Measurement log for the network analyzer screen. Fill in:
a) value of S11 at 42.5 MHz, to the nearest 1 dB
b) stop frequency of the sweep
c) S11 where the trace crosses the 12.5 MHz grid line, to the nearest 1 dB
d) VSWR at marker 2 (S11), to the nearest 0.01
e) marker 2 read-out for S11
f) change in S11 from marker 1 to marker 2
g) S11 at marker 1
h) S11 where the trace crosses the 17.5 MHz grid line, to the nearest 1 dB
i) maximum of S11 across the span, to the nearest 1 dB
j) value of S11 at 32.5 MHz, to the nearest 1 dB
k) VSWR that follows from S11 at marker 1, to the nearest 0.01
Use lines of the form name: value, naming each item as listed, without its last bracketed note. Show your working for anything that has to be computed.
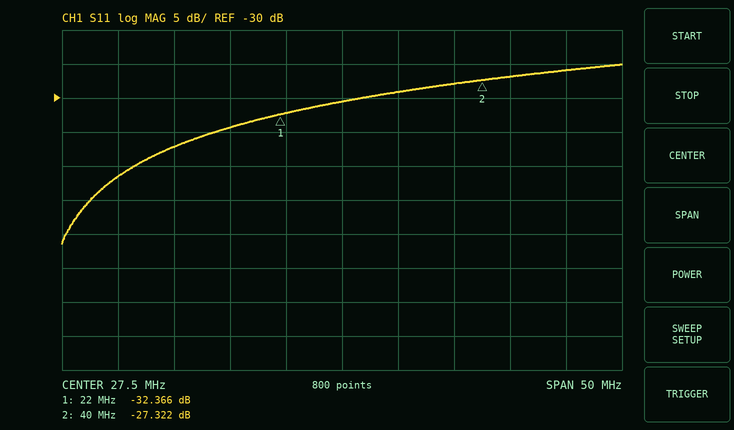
value of S11 at 42.5 MHz, to the nearest 1 dB: -27 dB
stop frequency of the sweep: 52.5 MHz
S11 where the trace crosses the 12.5 MHz grid line, to the nearest 1 dB: -37 dB
VSWR at marker 2 (S11), to the nearest 0.01: (1 + 0.0430)/(1 − 0.0430) ≈ 1.09
marker 2 read-out for S11: -27.322 dB
change in S11 from marker 1 to marker 2: -27.322 − (-32.366) = 5.044 dB
S11 at marker 1: -32.366 dB
S11 where the trace crosses the 17.5 MHz grid line, to the nearest 1 dB: -34 dB
maximum of S11 across the span, to the nearest 1 dB: -25 dB
value of S11 at 32.5 MHz, to the nearest 1 dB: -29 dB
VSWR that follows from S11 at marker 1, to the nearest 0.01: (1 + 0.0241)/(1 − 0.0241) ≈ 1.05
